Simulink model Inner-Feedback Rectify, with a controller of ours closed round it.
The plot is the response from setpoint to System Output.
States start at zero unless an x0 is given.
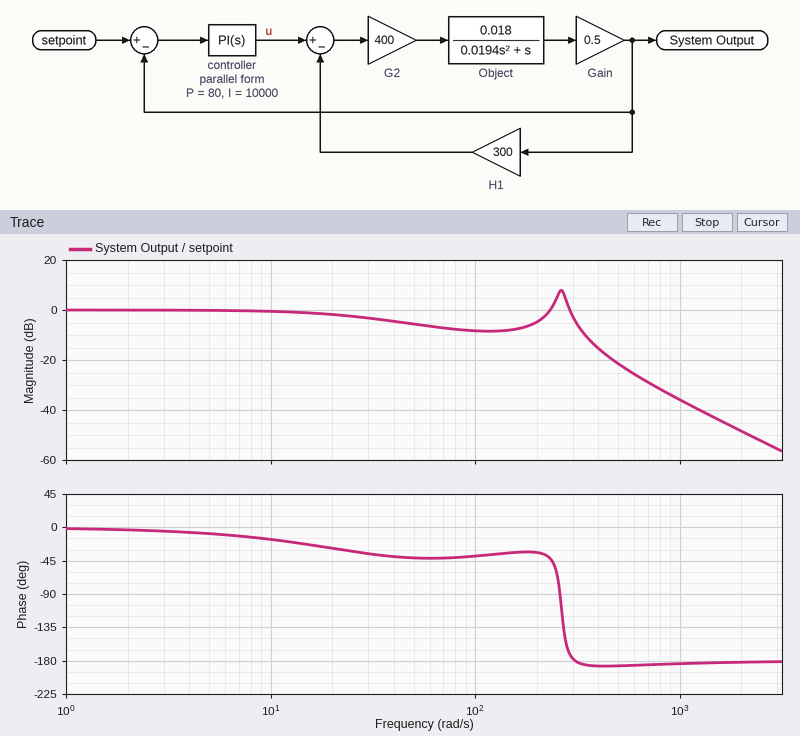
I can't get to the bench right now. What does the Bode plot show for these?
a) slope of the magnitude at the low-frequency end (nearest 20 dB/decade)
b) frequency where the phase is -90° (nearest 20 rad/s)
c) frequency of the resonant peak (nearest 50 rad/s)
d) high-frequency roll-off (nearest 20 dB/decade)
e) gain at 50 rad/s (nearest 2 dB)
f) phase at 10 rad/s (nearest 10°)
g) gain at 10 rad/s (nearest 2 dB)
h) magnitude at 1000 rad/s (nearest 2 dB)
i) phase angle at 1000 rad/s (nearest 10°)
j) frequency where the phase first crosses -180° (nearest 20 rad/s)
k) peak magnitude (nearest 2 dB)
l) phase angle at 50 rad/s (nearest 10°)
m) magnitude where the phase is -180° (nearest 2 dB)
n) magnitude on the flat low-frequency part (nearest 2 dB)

0 dB/decade
260 rad/s
250 rad/s
-40 dB/decade
-6 dB
-20°
0 dB
-36 dB
-180°
300 rad/s
8 dB
-40°
-4 dB
0 dB
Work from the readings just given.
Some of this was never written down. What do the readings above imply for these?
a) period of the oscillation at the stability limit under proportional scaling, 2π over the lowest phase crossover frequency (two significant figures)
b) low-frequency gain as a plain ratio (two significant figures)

0.021 s
1.0
